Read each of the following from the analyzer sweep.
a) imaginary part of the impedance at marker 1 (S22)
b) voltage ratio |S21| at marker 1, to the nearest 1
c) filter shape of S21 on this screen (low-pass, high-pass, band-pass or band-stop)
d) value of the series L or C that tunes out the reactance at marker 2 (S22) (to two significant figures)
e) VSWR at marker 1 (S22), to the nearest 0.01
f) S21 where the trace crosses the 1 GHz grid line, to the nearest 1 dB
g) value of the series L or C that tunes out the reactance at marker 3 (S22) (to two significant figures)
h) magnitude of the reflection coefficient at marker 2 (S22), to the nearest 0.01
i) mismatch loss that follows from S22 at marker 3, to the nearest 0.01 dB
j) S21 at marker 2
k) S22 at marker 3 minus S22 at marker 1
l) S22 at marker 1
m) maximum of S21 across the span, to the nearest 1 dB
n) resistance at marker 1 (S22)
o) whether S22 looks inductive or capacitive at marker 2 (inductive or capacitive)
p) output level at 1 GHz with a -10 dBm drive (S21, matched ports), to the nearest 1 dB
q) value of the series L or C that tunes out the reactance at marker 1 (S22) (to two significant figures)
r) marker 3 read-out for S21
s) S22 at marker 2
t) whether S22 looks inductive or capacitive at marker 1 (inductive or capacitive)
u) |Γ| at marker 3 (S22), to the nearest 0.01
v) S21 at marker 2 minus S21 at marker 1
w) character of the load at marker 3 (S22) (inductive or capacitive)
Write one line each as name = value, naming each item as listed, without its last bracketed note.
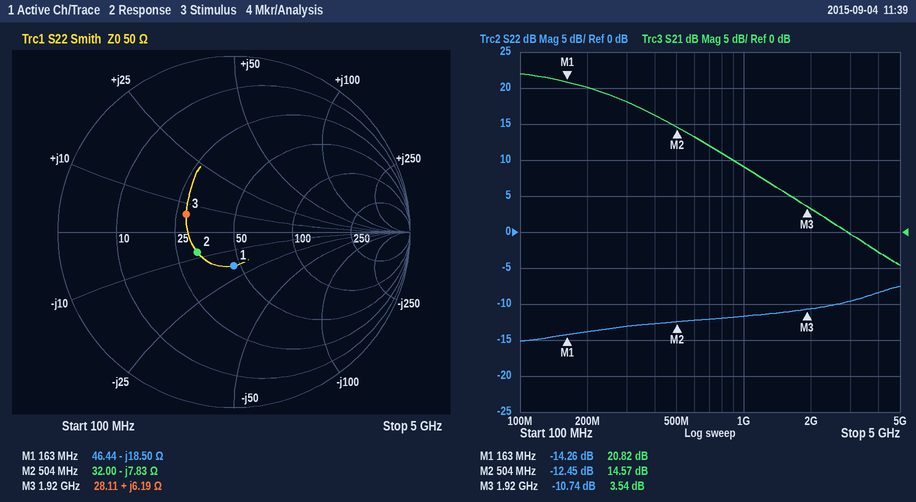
imaginary part of the impedance at marker 1 = -18.50 Ω
voltage ratio |S21| at marker 1, to the nearest 1 = 11
filter shape of S21 on this screen = low-pass
value of the series L or C that tunes out the reactance at marker 2 (S22) = 2.5 nH
VSWR at marker 1 (S22), to the nearest 0.01 = 1.48
S21 where the trace crosses the 1 GHz grid line, to the nearest 1 dB = 9 dB
value of the series L or C that tunes out the reactance at marker 3 (S22) = 13 pF
magnitude of the reflection coefficient at marker 2 (S22), to the nearest 0.01 = 0.24
mismatch loss that follows from S22 at marker 3, to the nearest 0.01 dB = 0.38 dB
S21 at marker 2 = 14.57 dB
S22 at marker 3 minus S22 at marker 1 = 3.52 dB
S22 at marker 1 = -14.26 dB
maximum of S21 across the span, to the nearest 1 dB = 22 dB
resistance at marker 1 = 46.44 Ω
whether S22 looks inductive or capacitive at marker 2 = capacitive
output level at 1 GHz with a -10 dBm drive (S21, matched ports), to the nearest 1 dB = -1 dBm
value of the series L or C that tunes out the reactance at marker 1 (S22) = 18 nH
marker 3 read-out for S21 = 3.54 dB
S22 at marker 2 = -12.45 dB
whether S22 looks inductive or capacitive at marker 1 = capacitive
|Γ| at marker 3 (S22), to the nearest 0.01 = 0.29
S21 at marker 2 minus S21 at marker 1 = -6.25 dB
character of the load at marker 3 (S22) = inductive
